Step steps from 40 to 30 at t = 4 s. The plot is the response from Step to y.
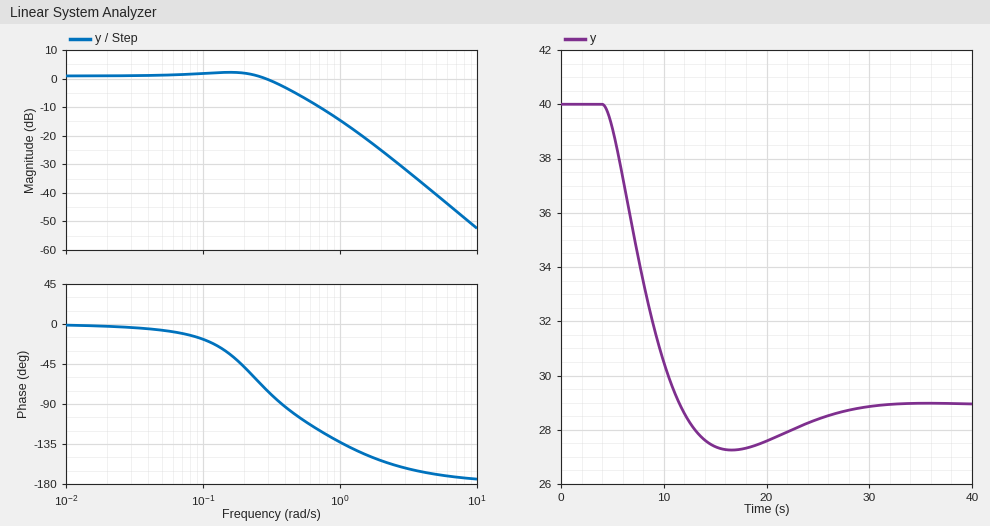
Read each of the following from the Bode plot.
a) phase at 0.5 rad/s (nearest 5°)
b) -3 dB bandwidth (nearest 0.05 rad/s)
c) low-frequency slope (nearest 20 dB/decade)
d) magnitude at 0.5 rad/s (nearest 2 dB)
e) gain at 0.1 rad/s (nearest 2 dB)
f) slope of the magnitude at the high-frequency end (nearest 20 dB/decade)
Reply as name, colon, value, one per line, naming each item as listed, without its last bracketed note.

phase at 0.5 rad/s: -105°
-3 dB bandwidth: 0.35 rad/s
low-frequency slope: 0 dB/decade
magnitude at 0.5 rad/s: -6 dB
gain at 0.1 rad/s: 2 dB
slope of the magnitude at the high-frequency end: -40 dB/decade
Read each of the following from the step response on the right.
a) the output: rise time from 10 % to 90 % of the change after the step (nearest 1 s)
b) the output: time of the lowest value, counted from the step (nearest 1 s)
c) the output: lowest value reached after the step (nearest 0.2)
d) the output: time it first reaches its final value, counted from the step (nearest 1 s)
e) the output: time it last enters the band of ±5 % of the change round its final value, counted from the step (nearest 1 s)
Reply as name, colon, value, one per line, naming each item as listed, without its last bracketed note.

the output: rise time from 10 % to 90 % of the change after the step: 5 s
the output: time of the lowest value, counted from the step: 13 s
the output: lowest value reached after the step: 27.2
the output: time it first reaches its final value, counted from the step: 8 s
the output: time it last enters the band of ±5 % of the change round its final value, counted from the step: 21 s
